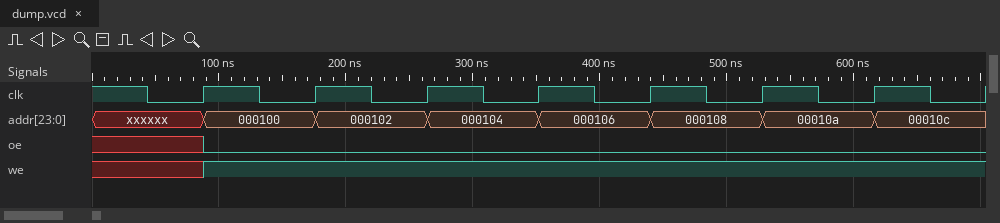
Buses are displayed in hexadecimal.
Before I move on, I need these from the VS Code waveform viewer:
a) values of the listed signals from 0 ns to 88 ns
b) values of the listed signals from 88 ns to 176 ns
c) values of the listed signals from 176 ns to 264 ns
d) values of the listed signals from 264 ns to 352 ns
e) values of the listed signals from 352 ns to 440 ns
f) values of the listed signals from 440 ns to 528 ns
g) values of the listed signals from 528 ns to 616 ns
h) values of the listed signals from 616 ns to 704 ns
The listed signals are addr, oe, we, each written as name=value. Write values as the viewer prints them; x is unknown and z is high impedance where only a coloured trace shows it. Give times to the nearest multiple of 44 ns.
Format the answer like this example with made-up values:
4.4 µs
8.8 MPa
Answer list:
addr=xxxxxx, oe=x, we=x
addr=000100, oe=0, we=1
addr=000102, oe=0, we=1
addr=000104, oe=0, we=1
addr=000106, oe=0, we=1
addr=000108, oe=0, we=1
addr=00010a, oe=0, we=1
addr=00010c, oe=0, we=1
